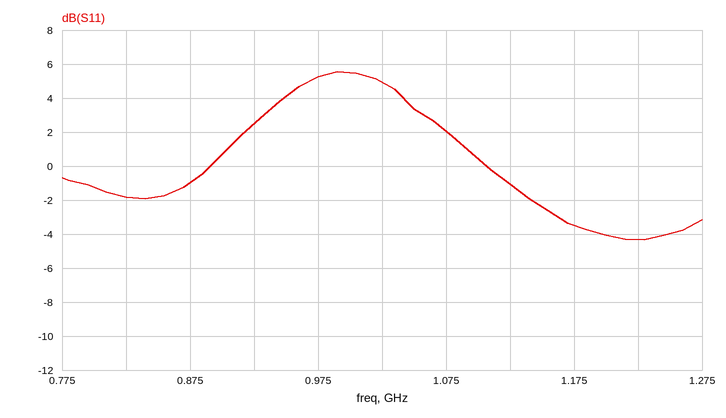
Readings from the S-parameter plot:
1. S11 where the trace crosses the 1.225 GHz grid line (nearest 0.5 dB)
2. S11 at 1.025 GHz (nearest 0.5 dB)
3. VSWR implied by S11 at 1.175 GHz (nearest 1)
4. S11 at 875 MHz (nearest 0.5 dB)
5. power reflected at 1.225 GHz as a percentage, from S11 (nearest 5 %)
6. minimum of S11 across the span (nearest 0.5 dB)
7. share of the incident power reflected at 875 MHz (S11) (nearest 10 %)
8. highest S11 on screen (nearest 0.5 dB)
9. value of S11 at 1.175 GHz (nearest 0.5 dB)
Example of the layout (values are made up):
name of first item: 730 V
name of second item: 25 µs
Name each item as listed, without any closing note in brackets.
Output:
S11 where the trace crosses the 1.225 GHz grid line: -4.5 dB
S11 at 1.025 GHz: 5.0 dB
VSWR implied by S11 at 1.175 GHz: 5
S11 at 875 MHz: -1.0 dB
power reflected at 1.225 GHz as a percentage, from S11: 35 %
minimum of S11 across the span: -4.5 dB
share of the incident power reflected at 875 MHz (S11): 80 %
highest S11 on screen: 5.5 dB
value of S11 at 1.175 GHz: -3.5 dB
